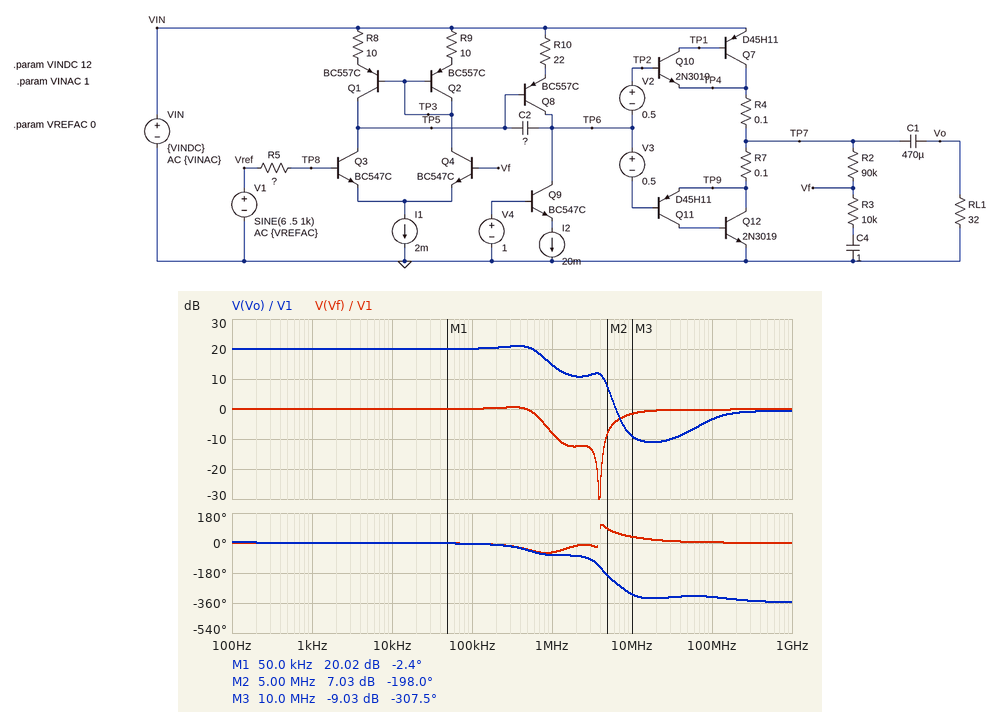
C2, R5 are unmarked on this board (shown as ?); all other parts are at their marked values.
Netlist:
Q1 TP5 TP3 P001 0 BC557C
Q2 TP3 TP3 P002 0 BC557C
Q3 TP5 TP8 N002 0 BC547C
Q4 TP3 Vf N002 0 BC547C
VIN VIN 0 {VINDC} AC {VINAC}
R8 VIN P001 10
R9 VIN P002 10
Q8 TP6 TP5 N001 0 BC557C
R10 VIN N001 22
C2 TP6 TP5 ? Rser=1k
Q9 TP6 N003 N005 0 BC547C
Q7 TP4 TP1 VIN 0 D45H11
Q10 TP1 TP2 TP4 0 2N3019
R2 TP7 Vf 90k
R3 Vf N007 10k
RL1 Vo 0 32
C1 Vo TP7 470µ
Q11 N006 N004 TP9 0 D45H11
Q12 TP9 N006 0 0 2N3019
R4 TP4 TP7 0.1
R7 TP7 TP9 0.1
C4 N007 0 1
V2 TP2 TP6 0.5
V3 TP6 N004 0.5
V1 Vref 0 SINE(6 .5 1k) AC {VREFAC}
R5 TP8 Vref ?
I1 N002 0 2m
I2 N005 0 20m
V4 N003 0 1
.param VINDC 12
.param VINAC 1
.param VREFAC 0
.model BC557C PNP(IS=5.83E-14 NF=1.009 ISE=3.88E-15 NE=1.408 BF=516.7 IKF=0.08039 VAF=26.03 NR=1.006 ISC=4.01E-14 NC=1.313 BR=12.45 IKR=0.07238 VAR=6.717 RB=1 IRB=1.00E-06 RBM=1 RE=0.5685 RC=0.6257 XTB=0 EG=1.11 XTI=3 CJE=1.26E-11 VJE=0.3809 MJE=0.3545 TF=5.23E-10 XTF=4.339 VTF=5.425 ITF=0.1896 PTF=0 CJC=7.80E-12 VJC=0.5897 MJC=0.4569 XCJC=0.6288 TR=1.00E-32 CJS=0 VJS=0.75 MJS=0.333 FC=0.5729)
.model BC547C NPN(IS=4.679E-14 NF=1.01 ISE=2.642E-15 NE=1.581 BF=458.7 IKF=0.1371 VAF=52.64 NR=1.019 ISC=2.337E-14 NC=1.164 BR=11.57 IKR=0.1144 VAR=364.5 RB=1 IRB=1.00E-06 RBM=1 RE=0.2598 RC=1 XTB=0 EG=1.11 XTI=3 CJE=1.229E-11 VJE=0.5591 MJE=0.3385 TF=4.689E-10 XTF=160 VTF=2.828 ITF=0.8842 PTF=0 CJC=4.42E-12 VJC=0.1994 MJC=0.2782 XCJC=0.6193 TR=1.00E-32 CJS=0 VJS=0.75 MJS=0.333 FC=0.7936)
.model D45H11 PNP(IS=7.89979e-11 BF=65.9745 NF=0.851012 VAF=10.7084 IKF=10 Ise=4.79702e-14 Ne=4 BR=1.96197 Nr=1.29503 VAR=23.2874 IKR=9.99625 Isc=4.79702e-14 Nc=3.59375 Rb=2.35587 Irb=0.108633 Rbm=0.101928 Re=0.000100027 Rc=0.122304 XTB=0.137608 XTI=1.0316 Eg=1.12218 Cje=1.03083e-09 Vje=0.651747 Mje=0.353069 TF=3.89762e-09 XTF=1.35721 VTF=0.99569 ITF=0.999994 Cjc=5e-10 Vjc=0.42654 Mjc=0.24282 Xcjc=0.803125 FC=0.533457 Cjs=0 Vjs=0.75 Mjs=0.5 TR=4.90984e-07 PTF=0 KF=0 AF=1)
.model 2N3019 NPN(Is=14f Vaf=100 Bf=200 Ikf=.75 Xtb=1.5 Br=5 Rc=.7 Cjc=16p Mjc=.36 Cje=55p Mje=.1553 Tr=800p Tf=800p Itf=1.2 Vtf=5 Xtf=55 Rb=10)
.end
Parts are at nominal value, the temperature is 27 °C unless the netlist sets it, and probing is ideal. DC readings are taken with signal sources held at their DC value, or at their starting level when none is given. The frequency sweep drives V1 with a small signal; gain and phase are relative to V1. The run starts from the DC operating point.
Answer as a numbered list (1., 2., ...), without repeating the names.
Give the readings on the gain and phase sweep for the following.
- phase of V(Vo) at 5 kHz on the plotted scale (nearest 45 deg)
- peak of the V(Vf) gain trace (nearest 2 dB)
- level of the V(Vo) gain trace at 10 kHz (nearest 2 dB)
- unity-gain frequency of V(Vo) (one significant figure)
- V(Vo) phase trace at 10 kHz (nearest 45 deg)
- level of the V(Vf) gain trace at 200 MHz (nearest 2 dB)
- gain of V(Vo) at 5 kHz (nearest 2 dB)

1. 0 deg
2. 0 dB
3. 20 dB
4. 6 MHz
5. 0 deg
6. 0 dB
7. 20 dB
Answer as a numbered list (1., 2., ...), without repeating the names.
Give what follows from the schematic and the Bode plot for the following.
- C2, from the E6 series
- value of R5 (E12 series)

1. 150 pF
2. 56 kΩ
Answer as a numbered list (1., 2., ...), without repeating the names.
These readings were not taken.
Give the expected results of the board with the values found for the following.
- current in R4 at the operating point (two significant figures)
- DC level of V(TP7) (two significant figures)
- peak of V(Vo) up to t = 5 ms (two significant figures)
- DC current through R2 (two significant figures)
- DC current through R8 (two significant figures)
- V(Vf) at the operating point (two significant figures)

1. 95 mA
2. 6.1 V
3. 4.9 V
4. 1.9 µA
5. 980 µA
6. 5.9 V
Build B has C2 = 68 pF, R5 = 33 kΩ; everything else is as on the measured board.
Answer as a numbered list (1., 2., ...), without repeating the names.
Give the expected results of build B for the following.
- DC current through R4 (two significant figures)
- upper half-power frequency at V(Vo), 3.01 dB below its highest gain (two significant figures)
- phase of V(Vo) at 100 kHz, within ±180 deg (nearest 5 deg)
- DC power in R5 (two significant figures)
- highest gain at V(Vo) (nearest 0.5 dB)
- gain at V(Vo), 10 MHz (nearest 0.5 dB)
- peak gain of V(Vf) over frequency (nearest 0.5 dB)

1. 95 mA
2. 1.3 MHz
3. 0 deg
4. 140 nW
5. 24.5 dB
6. -9.5 dB
7. 3.0 dB
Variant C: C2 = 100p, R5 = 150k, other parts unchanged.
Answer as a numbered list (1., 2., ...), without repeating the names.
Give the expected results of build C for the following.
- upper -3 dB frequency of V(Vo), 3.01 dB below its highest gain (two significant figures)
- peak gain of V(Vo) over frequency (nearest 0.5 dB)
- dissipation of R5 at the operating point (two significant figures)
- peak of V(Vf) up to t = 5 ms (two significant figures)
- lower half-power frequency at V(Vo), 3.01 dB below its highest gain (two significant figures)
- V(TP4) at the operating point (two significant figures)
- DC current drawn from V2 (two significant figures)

1. 560 kHz
2. 20.5 dB
3. 640 nW
4. 6.2 V
5. 12 Hz
6. 5.9 V
7. 4.5 µA
